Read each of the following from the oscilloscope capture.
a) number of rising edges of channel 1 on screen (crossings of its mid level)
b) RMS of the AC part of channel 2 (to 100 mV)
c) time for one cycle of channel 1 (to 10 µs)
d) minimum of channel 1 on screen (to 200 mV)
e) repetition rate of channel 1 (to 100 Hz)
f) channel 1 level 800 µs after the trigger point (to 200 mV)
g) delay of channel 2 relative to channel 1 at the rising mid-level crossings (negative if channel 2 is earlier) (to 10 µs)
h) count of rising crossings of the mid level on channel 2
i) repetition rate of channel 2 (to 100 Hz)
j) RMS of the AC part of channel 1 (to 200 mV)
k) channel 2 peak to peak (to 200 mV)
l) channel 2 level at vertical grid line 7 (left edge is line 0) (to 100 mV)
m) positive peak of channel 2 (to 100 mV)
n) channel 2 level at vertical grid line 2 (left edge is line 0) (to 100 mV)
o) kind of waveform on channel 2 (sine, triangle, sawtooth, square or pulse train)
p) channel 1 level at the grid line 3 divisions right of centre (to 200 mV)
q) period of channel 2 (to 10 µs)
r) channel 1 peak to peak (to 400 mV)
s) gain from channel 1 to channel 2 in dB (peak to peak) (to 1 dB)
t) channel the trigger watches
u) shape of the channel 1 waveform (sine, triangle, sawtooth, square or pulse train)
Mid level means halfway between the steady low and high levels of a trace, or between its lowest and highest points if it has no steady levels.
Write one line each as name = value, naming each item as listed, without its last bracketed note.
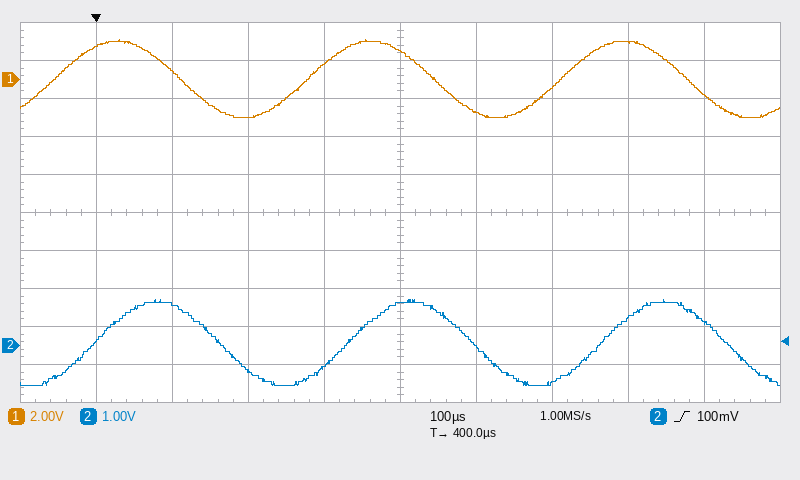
number of rising edges of channel 1 on screen = 3
RMS of the AC part of channel 2 = 800 mV
time for one cycle of channel 1 = 330 µs
minimum of channel 1 on screen = -2.0 V
repetition rate of channel 1 = 3.0 kHz
channel 1 level 800 µs after the trigger point = -800 mV
delay of channel 2 relative to channel 1 at the rising mid-level crossings (negative if channel 2 is earlier) = +50 µs
count of rising crossings of the mid level on channel 2 = 3
repetition rate of channel 2 = 3.0 kHz
RMS of the AC part of channel 1 = 1.4 V
channel 2 peak to peak = 2.2 V
channel 2 level at vertical grid line 7 (left edge is line 0) = -1.0 V
positive peak of channel 2 = 1.2 V
channel 2 level at vertical grid line 2 (left edge is line 0) = 1.1 V
kind of waveform on channel 2 = sine
channel 1 level at the grid line 3 divisions right of centre = 2.0 V
period of channel 2 = 330 µs
channel 1 peak to peak = 4.0 V
gain from channel 1 to channel 2 in dB (peak to peak) = -5 dB
channel the trigger watches = channel 2
shape of the channel 1 waveform = sine
